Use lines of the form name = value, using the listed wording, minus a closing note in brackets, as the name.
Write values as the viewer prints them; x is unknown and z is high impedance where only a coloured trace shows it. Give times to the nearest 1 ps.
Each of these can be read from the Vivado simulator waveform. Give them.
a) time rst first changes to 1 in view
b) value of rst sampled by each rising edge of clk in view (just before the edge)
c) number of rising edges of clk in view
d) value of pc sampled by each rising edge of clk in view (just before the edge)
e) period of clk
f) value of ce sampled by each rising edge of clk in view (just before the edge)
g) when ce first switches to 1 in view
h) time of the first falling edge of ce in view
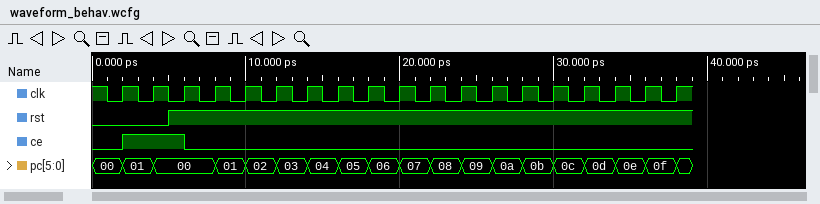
time rst first changes to 1 in view = 5 ps
value of rst sampled by each rising edge of clk in view = 0 0 1 1 1 1 1 1 1 1 1 1 1 1 1 1 1 1 1
number of rising edges of clk in view = 19
value of pc sampled by each rising edge of clk in view = 00, 01, 00, 00, 01, 02, 03, 04, 05, 06, 07, 08, 09, 0a, 0b, 0c, 0d, 0e, 0f
period of clk = 2 ps
value of ce sampled by each rising edge of clk in view = 0 1 1 0 0 0 0 0 0 0 0 0 0 0 0 0 0 0 0
when ce first switches to 1 in view = 2 ps
time of the first falling edge of ce in view = 6 ps
